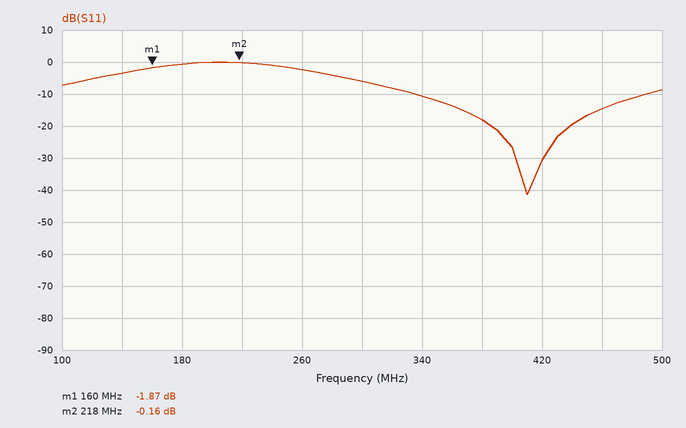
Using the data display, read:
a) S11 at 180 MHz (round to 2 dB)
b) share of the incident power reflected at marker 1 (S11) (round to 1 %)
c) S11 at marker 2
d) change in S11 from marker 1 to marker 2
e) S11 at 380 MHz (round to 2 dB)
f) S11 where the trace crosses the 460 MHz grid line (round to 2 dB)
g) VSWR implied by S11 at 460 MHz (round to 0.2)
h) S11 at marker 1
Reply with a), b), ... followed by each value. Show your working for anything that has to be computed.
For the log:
a) 0 dB
b) 10^(-1.87/10) ≈ 65 %
c) -0.16 dB
d) -0.16 − (-1.87) = 1.71 dB
e) -18 dB
f) -14 dB
g) |Γ| = 10^(-14/20) = 0.1995; VSWR = (1 + 0.1995)/(1 − 0.1995) ≈ 1.50, so 1.4 to the nearest 0.2
h) -1.87 dB
